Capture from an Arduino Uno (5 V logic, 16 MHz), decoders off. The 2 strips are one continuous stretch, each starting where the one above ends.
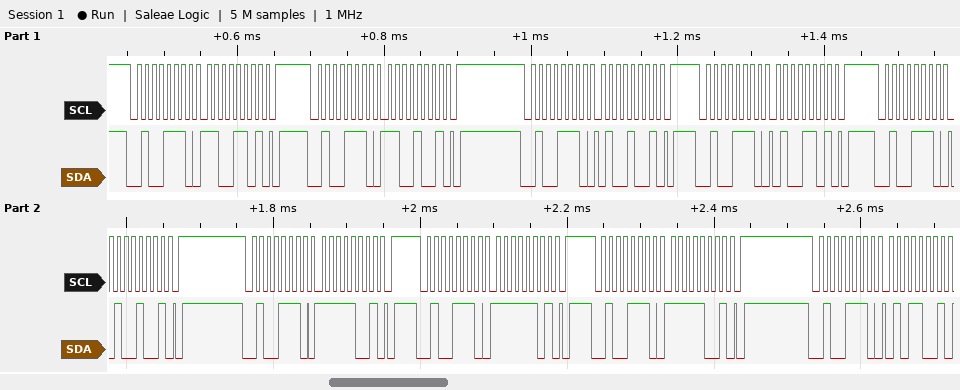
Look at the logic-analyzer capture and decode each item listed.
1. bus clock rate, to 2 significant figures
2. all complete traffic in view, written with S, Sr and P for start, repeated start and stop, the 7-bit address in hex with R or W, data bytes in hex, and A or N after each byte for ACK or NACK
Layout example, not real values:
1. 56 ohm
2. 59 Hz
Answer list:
1. 100 kHz
2. S 27W A CD A P S 27W A C9 A P S 27W A 49 A P S 27W A 4D A P S 27W A 49 A P S 27W A F9 A P S 27W A FD A P S 27W A F9 A P S 27W A 59 A
